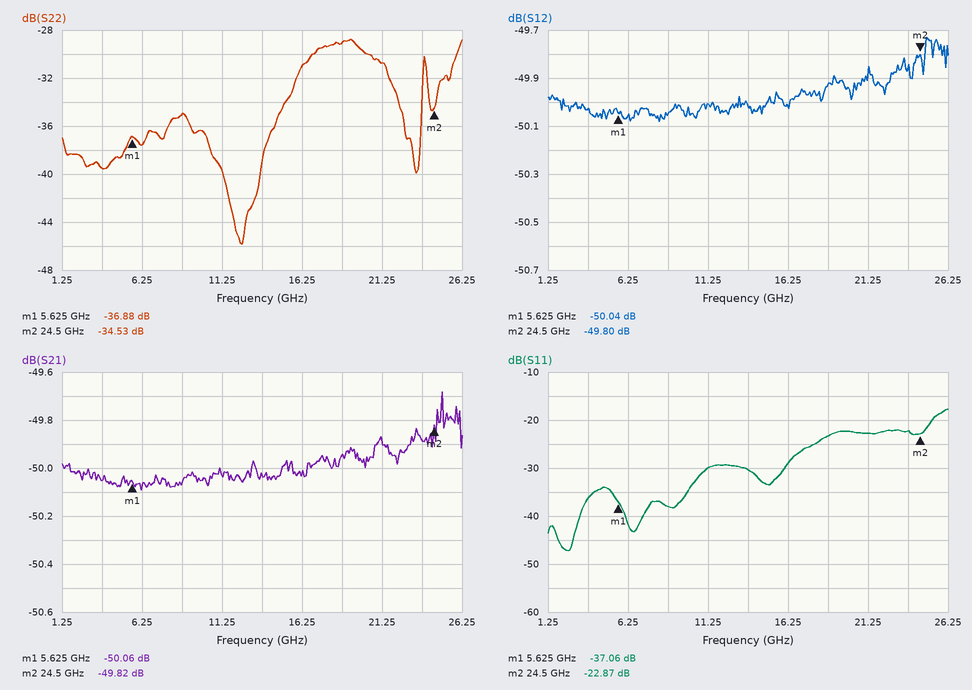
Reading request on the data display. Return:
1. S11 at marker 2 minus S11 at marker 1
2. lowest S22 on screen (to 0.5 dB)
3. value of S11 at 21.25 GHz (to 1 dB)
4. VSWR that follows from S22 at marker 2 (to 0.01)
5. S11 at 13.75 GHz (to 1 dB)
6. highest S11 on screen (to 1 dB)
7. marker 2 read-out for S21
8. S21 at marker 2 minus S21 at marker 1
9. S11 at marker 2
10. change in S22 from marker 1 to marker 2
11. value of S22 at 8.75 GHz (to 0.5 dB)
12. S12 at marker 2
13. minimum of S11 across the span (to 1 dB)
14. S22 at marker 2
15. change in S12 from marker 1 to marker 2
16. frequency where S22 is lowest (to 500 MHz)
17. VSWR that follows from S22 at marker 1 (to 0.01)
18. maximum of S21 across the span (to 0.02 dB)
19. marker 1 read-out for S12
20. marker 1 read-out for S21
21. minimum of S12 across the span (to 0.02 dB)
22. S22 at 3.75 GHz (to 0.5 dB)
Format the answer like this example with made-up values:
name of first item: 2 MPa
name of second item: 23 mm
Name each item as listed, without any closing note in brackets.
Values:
S11 at marker 2 minus S11 at marker 1: 14.19 dB
lowest S22 on screen: -46.0 dB
value of S11 at 21.25 GHz: -23 dB
VSWR that follows from S22 at marker 2: 1.04
S11 at 13.75 GHz: -30 dB
highest S11 on screen: -18 dB
marker 2 read-out for S21: -49.82 dB
S21 at marker 2 minus S21 at marker 1: 0.24 dB
S11 at marker 2: -22.87 dB
change in S22 from marker 1 to marker 2: 2.35 dB
value of S22 at 8.75 GHz: -35.0 dB
S12 at marker 2: -49.80 dB
minimum of S11 across the span: -47 dB
S22 at marker 2: -34.53 dB
change in S12 from marker 1 to marker 2: 0.24 dB
frequency where S22 is lowest: 12.5 GHz
VSWR that follows from S22 at marker 1: 1.03
maximum of S21 across the span: -49.68 dB
marker 1 read-out for S12: -50.04 dB
marker 1 read-out for S21: -50.06 dB
minimum of S12 across the span: -50.08 dB
S22 at 3.75 GHz: -39.5 dB
